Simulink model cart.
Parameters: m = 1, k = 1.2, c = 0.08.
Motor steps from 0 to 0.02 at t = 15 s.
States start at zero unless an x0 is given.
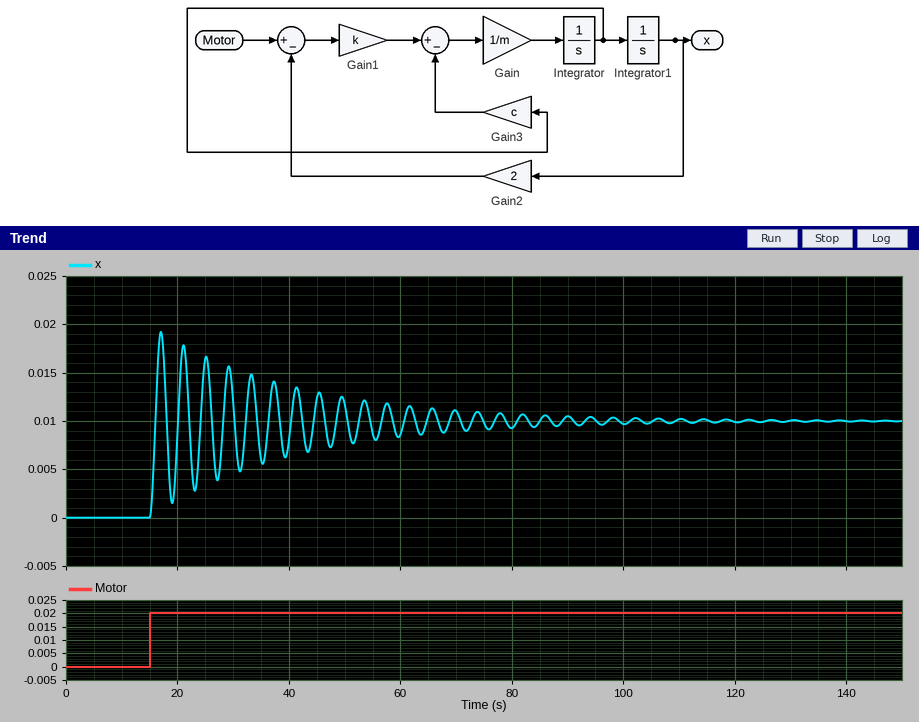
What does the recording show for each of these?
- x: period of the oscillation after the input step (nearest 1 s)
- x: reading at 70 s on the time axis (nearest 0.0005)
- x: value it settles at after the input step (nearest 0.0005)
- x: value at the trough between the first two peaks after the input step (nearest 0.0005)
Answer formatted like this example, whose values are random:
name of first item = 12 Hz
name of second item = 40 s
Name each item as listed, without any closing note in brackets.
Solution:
x: period of the oscillation after the input step = 4 s
x: reading at 70 s on the time axis = 0.0110
x: value it settles at after the input step = 0.0100
x: value at the trough between the first two peaks after the input step = 0.0015
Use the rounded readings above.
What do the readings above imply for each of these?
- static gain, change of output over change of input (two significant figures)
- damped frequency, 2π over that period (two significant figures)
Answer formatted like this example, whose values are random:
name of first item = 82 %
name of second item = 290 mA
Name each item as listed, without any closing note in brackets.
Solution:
static gain, change of output over change of input = 0.50
damped frequency, 2π over that period = 1.6 rad/s
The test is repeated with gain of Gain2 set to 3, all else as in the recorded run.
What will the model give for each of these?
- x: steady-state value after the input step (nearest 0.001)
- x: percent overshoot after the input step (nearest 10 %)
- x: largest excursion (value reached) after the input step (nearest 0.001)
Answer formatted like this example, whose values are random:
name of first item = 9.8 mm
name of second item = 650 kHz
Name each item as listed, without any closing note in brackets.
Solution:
x: steady-state value after the input step = 0.007
x: percent overshoot after the input step = 90 %
x: largest excursion (value reached) after the input step = 0.013
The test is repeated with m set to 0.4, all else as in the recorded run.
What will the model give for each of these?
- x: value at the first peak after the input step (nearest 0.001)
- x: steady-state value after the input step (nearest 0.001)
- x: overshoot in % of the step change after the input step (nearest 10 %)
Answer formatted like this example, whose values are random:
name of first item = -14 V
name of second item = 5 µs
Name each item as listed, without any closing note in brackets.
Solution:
x: value at the first peak after the input step = 0.019
x: steady-state value after the input step = 0.010
x: overshoot in % of the step change after the input step = 90 %
